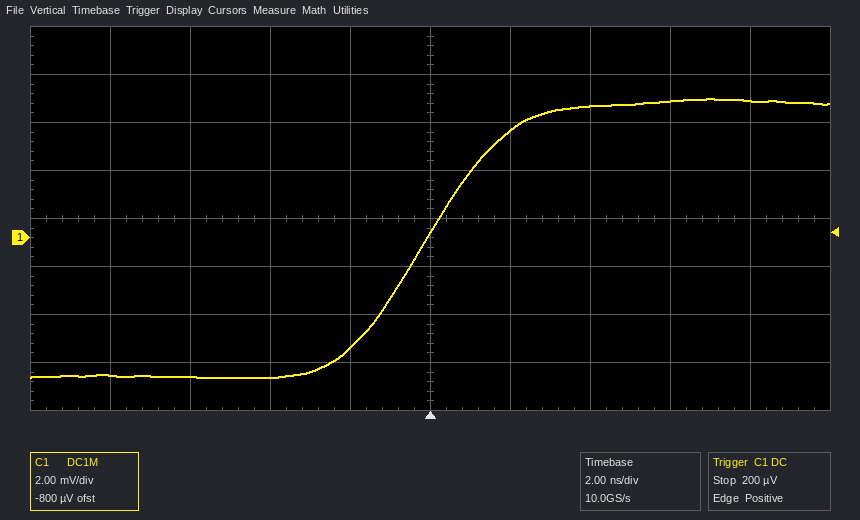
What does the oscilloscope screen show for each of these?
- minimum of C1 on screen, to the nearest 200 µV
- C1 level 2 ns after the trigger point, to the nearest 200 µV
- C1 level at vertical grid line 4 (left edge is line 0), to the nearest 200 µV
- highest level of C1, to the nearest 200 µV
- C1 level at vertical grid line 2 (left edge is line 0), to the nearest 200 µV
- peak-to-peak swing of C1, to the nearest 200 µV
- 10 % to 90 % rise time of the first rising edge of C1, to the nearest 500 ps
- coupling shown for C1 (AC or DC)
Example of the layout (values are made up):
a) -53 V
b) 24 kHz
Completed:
a) -5.8 mV
b) 4.4 mV
c) -4.6 mV
d) 5.8 mV
e) -5.8 mV
f) 11.6 mV
g) 4.0 ns
h) DC
